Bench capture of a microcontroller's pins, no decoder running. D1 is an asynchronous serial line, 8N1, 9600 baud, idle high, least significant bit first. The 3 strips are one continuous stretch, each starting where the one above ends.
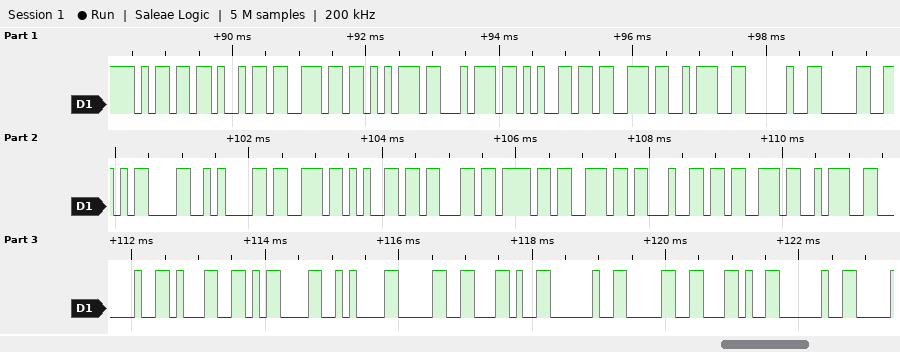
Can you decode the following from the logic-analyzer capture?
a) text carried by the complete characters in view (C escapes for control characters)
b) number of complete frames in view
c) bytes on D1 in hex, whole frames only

"minutes: 0\r\nseconds: 1\r\n0, 0, "
30
6D 69 6E 75 74 65 73 3A 20 30 0D 0A 73 65 63 6F 6E 64 73 3A 20 31 0D 0A 30 2C 20 30 2C 20
